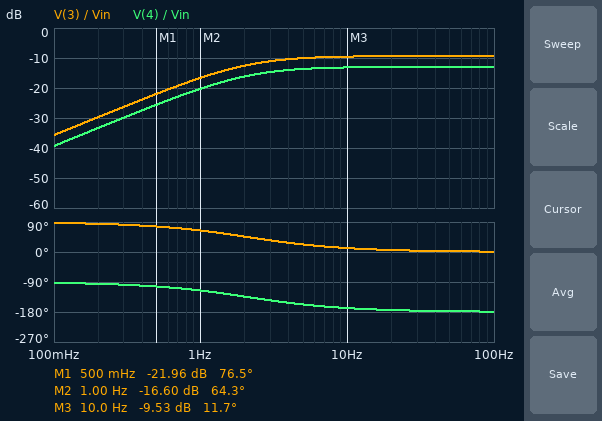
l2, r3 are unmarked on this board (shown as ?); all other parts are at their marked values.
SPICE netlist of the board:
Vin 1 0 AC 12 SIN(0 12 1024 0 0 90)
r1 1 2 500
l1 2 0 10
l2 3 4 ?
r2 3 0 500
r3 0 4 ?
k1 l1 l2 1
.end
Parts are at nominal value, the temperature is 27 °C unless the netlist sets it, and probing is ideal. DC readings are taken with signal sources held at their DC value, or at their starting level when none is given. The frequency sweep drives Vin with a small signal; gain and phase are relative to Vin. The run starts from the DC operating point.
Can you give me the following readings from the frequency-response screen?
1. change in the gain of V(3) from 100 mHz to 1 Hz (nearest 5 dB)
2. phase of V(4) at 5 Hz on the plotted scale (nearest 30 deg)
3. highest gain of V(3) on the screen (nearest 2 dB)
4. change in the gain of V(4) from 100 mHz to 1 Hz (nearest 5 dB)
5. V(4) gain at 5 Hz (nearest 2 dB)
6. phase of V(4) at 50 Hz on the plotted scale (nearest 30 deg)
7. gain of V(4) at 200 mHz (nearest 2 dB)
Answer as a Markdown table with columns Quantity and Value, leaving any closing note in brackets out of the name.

| Quantity | Value |
|---|---|
| change in the gain of V(3) from 100 mHz to 1 Hz | 20 dB |
| phase of V(4) at 5 Hz on the plotted scale | -150 deg |
| highest gain of V(3) on the screen | -10 dB |
| change in the gain of V(4) from 100 mHz to 1 Hz | 20 dB |
| V(4) gain at 5 Hz | -14 dB |
| phase of V(4) at 50 Hz on the plotted scale | -180 deg |
| gain of V(4) at 200 mHz | -34 dB |
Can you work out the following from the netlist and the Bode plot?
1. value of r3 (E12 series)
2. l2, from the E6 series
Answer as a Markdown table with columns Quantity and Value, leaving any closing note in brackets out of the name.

| Quantity | Value |
|---|---|
| value of r3 | 330 Ω |
| l2, from the E6 series | 47 H |
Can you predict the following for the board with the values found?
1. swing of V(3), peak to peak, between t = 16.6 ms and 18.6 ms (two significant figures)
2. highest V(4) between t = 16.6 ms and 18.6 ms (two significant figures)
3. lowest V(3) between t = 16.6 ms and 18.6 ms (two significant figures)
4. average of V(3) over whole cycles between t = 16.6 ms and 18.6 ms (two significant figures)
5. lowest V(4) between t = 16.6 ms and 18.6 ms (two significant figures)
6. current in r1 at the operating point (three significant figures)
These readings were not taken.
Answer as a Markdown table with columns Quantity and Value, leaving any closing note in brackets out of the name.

| Quantity | Value |
|---|---|
| swing of V(3), peak to peak, between t = 16.6 ms and 18.6 ms | 8.2 V |
| highest V(4) between t = 16.6 ms and 18.6 ms | 4.9 V |
| lowest V(3) between t = 16.6 ms and 18.6 ms | -7.4 V |
| average of V(3) over whole cycles between t = 16.6 ms and 18.6 ms | -3.3 V |
| lowest V(4) between t = 16.6 ms and 18.6 ms | -580 mV |
| current in r1 at the operating point | 24.0 mA |
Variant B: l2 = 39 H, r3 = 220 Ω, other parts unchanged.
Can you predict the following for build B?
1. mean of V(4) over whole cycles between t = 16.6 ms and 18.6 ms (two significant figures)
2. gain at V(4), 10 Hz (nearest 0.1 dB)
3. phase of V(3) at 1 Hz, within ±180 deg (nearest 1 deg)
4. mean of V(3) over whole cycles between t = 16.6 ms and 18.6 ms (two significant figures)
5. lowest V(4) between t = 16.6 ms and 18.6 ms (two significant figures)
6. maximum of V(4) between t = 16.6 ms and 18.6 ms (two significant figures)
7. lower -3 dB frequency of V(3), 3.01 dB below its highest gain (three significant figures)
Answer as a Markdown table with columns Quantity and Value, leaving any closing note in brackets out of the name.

| Quantity | Value |
|---|---|
| mean of V(4) over whole cycles between t = 16.6 ms and 18.6 ms | 1.5 V |
| gain at V(4), 10 Hz | -16.0 dB |
| phase of V(3) at 1 Hz, within ±180 deg | 65 deg |
| mean of V(3) over whole cycles between t = 16.6 ms and 18.6 ms | -3.5 V |
| lowest V(4) between t = 16.6 ms and 18.6 ms | -430 mV |
| maximum of V(4) between t = 16.6 ms and 18.6 ms | 3.5 V |
| lower -3 dB frequency of V(3), 3.01 dB below its highest gain | 2.15 Hz |
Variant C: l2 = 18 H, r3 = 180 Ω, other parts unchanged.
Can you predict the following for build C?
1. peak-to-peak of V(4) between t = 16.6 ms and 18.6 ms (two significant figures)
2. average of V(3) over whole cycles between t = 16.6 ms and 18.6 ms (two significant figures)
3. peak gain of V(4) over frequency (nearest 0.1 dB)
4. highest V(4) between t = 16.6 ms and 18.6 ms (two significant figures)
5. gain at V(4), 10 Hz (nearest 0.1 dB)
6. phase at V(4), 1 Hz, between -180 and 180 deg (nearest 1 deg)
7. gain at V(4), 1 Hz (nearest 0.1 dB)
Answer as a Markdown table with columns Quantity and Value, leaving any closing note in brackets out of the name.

| Quantity | Value |
|---|---|
| peak-to-peak of V(4) between t = 16.6 ms and 18.6 ms | 3.7 V |
| average of V(3) over whole cycles between t = 16.6 ms and 18.6 ms | -3.5 V |
| peak gain of V(4) over frequency | -16.3 dB |
| highest V(4) between t = 16.6 ms and 18.6 ms | 3.1 V |
| gain at V(4), 10 Hz | -16.8 dB |
| phase at V(4), 1 Hz, between -180 and 180 deg | -106 deg |
| gain at V(4), 1 Hz | -27.4 dB |
